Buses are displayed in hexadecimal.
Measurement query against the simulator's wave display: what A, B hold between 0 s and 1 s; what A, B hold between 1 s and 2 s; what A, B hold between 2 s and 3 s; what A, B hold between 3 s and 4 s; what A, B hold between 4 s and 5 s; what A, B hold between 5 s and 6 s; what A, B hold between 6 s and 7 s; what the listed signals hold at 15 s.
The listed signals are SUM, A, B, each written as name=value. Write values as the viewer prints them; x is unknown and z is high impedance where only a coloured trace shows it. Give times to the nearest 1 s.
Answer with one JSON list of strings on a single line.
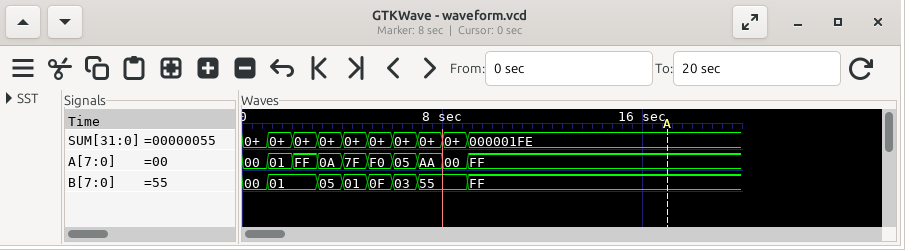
["A=00, B=00", "A=01, B=01", "A=FF, B=01", "A=0A, B=05", "A=7F, B=01", "A=F0, B=0F", "A=05, B=03", "SUM=000001FE, A=FF, B=FF"]
